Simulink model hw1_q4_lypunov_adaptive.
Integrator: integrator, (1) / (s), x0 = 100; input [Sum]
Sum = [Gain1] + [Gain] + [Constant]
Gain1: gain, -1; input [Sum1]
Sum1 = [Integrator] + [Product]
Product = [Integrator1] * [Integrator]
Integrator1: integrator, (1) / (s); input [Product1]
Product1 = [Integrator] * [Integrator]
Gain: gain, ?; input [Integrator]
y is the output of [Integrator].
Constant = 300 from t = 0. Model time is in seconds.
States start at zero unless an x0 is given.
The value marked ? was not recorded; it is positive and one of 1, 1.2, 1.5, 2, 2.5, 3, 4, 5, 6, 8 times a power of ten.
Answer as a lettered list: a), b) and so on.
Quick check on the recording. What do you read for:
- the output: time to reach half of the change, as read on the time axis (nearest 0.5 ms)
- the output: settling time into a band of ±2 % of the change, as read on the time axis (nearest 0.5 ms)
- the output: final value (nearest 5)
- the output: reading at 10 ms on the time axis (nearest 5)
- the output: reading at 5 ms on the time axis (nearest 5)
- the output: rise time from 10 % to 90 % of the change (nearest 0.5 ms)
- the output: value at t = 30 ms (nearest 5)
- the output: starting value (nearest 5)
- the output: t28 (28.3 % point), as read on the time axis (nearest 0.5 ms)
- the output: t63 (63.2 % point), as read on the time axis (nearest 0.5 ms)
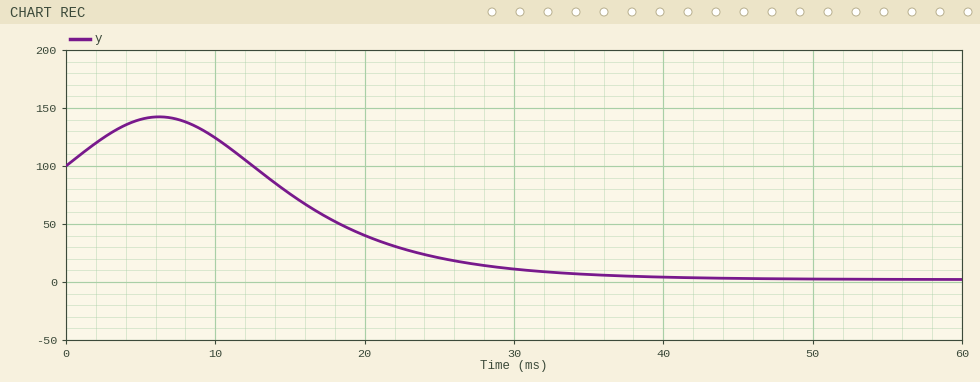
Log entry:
a) 18.0 ms
b) 40.5 ms
c) 0
d) 125
e) 140
f) 16.0 ms
g) 10
h) 100
i) 15.5 ms
j) 20.5 ms
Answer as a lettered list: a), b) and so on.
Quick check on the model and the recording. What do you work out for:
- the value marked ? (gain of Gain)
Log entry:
a) 100
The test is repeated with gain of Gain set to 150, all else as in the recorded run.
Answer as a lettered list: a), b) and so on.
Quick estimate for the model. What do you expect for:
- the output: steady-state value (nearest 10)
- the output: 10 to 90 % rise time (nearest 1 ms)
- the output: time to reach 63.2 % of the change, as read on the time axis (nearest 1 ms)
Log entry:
a) 0
b) 12 ms
c) 19 ms
